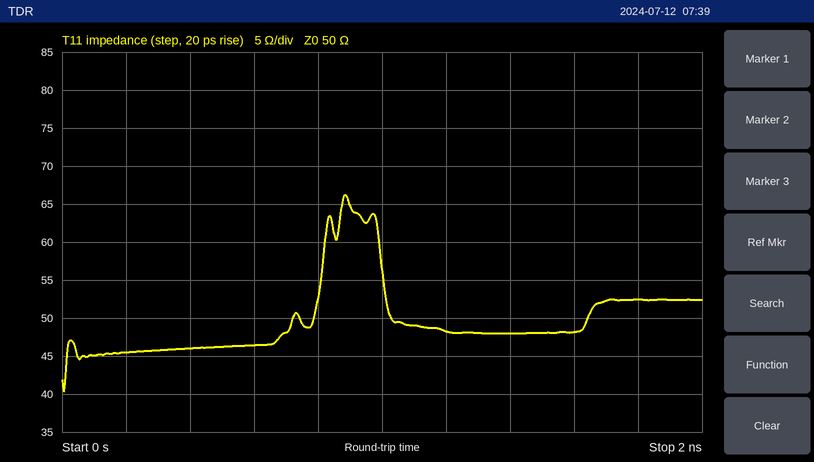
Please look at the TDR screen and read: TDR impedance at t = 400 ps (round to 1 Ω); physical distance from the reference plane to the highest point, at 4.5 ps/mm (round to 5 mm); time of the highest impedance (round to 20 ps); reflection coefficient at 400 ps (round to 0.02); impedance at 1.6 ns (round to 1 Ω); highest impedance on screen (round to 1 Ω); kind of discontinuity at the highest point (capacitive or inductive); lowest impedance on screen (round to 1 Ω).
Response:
46 Ω
100 mm
880 ps
-0.04
48 Ω
66 Ω
inductive
40 Ω
